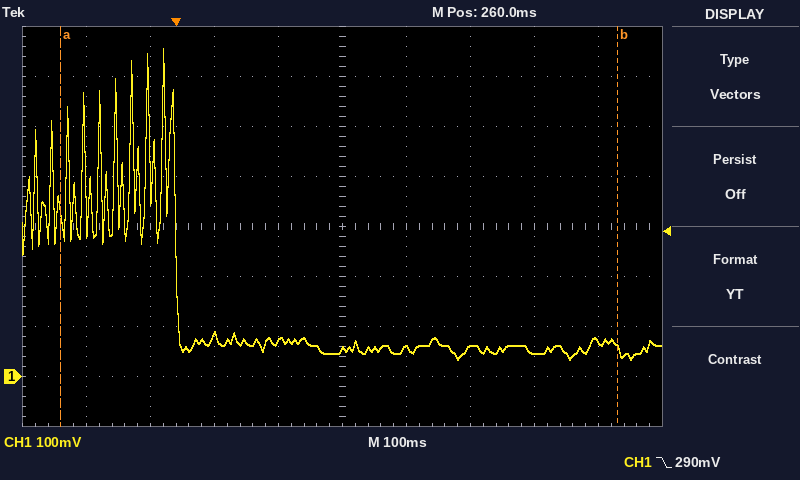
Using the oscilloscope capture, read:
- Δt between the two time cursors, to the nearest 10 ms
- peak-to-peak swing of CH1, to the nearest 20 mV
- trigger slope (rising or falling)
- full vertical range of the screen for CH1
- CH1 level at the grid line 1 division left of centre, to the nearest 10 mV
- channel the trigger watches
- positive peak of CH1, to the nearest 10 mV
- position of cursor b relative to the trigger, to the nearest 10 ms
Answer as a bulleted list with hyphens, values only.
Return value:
- 870 ms
- 620 mV
- falling
- 800 mV
- 70 mV
- CH1
- 660 mV
- +690 ms
